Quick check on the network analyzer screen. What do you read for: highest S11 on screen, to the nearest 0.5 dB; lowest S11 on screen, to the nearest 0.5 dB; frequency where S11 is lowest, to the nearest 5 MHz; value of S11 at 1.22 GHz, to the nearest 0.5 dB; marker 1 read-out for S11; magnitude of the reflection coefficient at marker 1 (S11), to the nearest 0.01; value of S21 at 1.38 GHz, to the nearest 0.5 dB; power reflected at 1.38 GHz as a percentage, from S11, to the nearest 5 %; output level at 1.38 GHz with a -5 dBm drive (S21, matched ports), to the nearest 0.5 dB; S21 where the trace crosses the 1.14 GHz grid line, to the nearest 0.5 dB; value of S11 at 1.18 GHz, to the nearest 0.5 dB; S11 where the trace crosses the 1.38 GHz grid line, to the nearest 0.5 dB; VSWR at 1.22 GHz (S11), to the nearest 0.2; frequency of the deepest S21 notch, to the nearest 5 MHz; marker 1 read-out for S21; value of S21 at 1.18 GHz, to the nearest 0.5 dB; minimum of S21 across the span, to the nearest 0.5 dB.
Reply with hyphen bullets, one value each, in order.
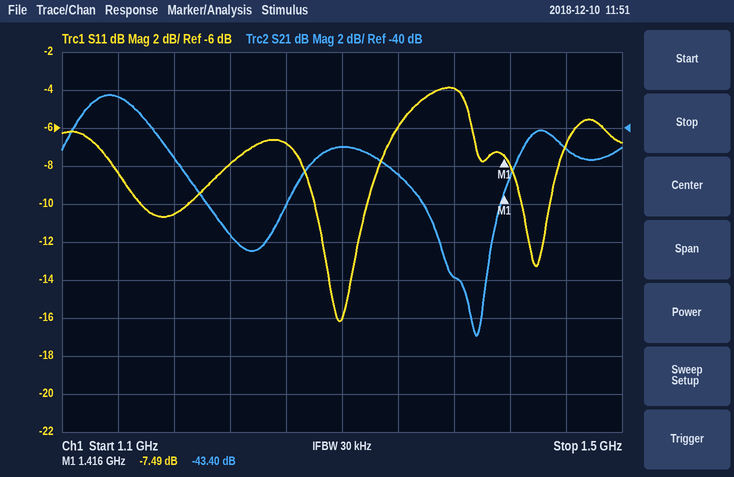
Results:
- -4.0 dB
- -16.0 dB
- 1.300 GHz
- -8.0 dB
- -7.49 dB
- 0.42
- -48.0 dB
- 40 %
- -53.0 dBm
- -38.5 dB
- -10.5 dB
- -4.0 dB
- 2.4
- 1.395 GHz
- -43.40 dB
- -41.5 dB
- -51.0 dB
